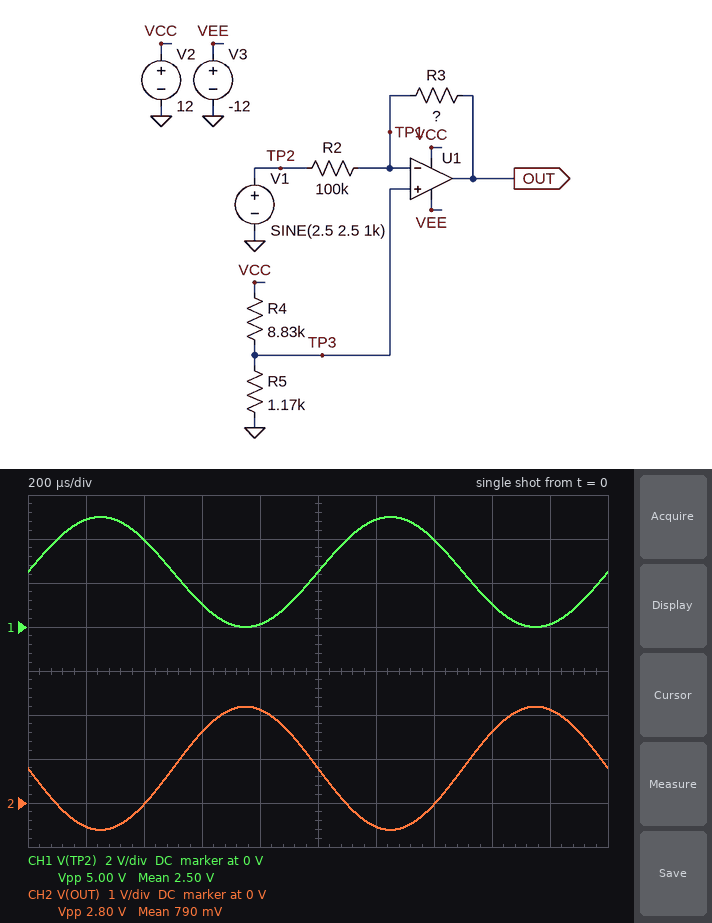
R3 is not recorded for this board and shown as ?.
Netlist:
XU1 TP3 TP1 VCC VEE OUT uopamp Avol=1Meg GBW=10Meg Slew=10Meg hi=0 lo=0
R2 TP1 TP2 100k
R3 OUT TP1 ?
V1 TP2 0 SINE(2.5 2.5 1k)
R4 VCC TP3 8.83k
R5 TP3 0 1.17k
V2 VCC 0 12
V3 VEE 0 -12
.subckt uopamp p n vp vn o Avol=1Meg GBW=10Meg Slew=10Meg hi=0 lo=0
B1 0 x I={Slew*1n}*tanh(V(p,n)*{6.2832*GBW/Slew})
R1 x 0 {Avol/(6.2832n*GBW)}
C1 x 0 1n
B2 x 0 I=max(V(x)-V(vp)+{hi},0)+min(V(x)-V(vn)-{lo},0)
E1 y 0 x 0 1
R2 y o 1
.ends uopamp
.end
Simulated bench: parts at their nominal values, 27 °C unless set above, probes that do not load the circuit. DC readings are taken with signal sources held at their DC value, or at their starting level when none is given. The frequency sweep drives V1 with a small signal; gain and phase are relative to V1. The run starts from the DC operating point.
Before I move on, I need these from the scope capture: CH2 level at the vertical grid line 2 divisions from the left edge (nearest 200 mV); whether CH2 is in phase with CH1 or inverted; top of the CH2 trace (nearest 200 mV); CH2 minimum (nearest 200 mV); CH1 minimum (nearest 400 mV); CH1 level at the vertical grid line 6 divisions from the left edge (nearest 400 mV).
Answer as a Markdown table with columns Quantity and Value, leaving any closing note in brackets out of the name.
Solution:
| Quantity | Value |
|---|---|
| CH2 level at the vertical grid line 2 divisions from the left edge | 0 V |
| whether CH2 is in phase with CH1 or inverted | inverted |
| top of the CH2 trace | 2.2 V |
| CH2 minimum | -600 mV |
| CH1 minimum | 0 V |
| CH1 level at the vertical grid line 6 divisions from the left edge | 4.8 V |
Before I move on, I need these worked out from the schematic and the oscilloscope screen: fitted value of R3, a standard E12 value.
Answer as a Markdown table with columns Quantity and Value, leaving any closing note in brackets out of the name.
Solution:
| Quantity | Value |
|---|---|
| fitted value of R3, a standard E12 value | 56 kΩ |
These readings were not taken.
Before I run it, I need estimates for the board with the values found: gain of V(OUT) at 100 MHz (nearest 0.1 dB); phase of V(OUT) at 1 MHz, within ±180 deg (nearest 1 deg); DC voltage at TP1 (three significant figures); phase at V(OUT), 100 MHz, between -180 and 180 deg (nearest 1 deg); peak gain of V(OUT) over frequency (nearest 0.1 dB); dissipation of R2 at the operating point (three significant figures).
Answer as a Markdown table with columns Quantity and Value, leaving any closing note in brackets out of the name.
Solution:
| Quantity | Value |
|---|---|
| gain of V(OUT) at 100 MHz | -28.9 dB |
| phase of V(OUT) at 1 MHz, within ±180 deg | 171 deg |
| DC voltage at TP1 | 1.40 V |
| phase at V(OUT), 100 MHz, between -180 and 180 deg | 94 deg |
| peak gain of V(OUT) over frequency | -5.0 dB |
| dissipation of R2 at the operating point | 12.0 µW |
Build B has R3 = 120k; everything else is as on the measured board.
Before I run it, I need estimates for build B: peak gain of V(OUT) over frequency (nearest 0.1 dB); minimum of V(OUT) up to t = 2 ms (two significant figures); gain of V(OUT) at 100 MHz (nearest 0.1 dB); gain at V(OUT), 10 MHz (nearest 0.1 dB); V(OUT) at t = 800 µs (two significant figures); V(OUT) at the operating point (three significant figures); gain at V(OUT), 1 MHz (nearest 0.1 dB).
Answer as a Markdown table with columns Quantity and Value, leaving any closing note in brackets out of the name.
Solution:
| Quantity | Value |
|---|---|
| peak gain of V(OUT) over frequency | 1.6 dB |
| minimum of V(OUT) up to t = 2 ms | -2.9 V |
| gain of V(OUT) at 100 MHz | -25.3 dB |
| gain at V(OUT), 10 MHz | -6.1 dB |
| V(OUT) at t = 800 µs | 2.9 V |
| V(OUT) at the operating point | 88.8 mV |
| gain at V(OUT), 1 MHz | 1.4 dB |
